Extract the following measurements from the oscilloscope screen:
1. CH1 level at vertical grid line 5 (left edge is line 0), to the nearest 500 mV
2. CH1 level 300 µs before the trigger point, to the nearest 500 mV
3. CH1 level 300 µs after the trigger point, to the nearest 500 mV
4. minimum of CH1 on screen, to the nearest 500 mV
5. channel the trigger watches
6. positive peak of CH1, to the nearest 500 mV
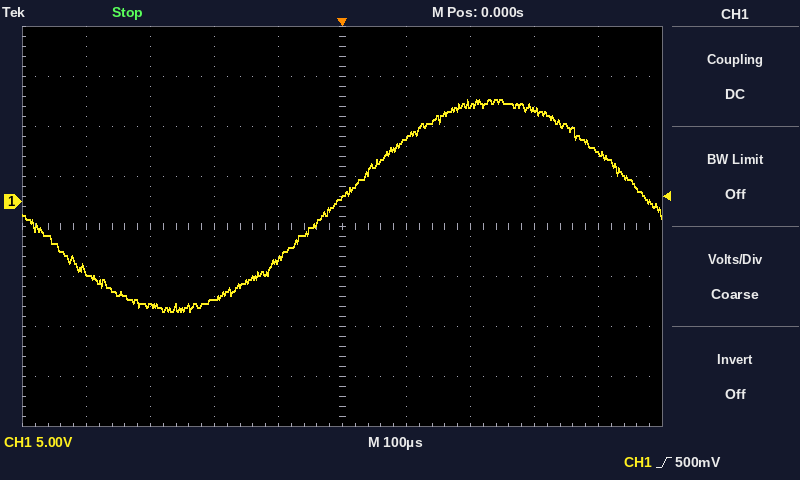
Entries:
500 mV
-10.5 V
9.0 V
-11.0 V
CH1
10.0 V
